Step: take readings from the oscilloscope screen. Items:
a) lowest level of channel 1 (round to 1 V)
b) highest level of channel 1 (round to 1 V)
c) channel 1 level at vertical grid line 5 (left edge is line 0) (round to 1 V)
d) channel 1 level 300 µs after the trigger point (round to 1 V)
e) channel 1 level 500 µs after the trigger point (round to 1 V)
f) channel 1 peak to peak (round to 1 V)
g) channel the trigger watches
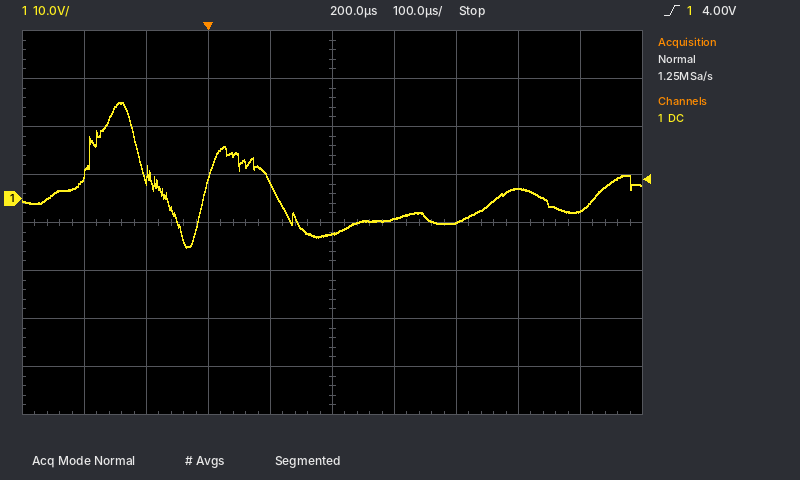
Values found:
-10 V
20 V
-7 V
-4 V
2 V
30 V
channel 1
